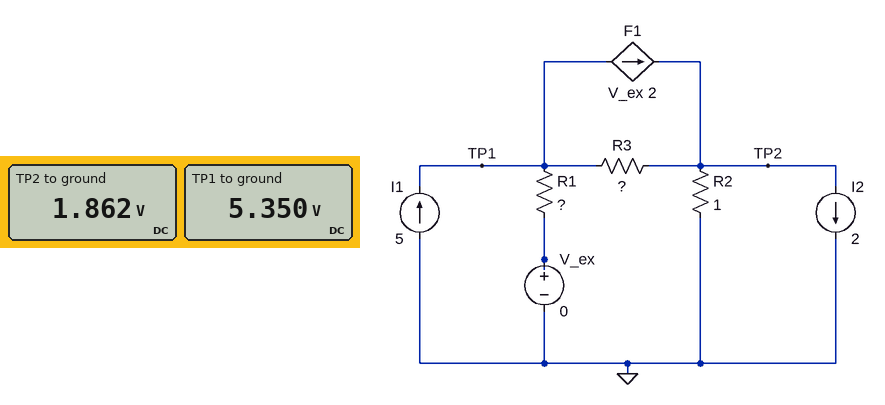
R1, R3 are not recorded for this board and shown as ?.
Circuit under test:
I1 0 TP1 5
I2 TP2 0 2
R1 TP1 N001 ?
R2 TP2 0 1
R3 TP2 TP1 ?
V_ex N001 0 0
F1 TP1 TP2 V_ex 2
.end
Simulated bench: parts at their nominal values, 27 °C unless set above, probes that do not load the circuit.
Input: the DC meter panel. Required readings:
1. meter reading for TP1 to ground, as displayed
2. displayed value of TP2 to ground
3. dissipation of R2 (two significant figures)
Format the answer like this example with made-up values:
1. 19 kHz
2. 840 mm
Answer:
1. 5.350 V
2. 1.862 V
3. 3.5 W
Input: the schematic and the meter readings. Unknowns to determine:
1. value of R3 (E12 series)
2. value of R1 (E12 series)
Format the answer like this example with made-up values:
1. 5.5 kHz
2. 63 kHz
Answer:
1. 2.2 Ω
2. 4.7 Ω
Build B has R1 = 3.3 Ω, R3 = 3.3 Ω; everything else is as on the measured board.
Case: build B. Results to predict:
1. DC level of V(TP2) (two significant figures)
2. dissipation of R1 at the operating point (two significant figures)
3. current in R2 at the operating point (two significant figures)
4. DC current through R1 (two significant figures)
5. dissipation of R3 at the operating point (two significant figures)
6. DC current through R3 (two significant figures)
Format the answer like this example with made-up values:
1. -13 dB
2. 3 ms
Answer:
1. 1.6 V
2. 6.2 W
3. 1.6 A
4. 1.4 A
5. 2.6 W
6. 880 mA
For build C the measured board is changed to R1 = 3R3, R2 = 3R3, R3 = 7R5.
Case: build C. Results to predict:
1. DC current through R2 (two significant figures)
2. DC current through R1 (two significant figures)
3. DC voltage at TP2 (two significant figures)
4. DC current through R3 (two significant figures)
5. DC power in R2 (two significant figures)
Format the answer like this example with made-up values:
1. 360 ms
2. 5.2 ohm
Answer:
1. 1.4 A
2. 1.6 A
3. 4.5 V
4. 110 mA
5. 6.2 W
